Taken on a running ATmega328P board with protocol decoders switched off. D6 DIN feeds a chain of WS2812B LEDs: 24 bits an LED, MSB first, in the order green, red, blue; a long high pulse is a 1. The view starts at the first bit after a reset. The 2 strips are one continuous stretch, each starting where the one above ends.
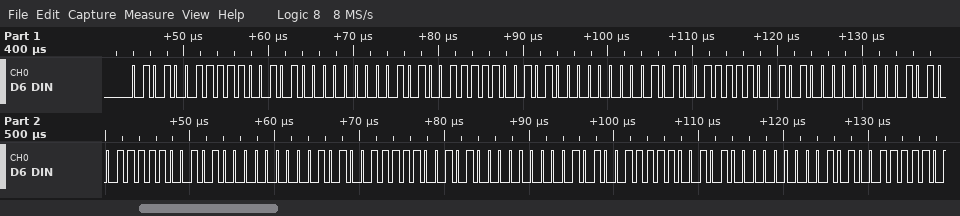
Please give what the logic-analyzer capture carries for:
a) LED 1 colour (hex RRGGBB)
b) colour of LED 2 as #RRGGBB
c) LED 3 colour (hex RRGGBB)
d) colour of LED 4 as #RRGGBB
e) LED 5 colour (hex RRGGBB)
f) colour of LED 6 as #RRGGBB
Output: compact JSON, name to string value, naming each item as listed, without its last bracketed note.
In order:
{"LED 1 colour": "#E55300", "colour of LED 2 as #RRGGBB": "#E55300", "LED 3 colour": "#E55300", "colour of LED 4 as #RRGGBB": "#E55300", "LED 5 colour": "#E55300", "colour of LED 6 as #RRGGBB": "#E55300"}
